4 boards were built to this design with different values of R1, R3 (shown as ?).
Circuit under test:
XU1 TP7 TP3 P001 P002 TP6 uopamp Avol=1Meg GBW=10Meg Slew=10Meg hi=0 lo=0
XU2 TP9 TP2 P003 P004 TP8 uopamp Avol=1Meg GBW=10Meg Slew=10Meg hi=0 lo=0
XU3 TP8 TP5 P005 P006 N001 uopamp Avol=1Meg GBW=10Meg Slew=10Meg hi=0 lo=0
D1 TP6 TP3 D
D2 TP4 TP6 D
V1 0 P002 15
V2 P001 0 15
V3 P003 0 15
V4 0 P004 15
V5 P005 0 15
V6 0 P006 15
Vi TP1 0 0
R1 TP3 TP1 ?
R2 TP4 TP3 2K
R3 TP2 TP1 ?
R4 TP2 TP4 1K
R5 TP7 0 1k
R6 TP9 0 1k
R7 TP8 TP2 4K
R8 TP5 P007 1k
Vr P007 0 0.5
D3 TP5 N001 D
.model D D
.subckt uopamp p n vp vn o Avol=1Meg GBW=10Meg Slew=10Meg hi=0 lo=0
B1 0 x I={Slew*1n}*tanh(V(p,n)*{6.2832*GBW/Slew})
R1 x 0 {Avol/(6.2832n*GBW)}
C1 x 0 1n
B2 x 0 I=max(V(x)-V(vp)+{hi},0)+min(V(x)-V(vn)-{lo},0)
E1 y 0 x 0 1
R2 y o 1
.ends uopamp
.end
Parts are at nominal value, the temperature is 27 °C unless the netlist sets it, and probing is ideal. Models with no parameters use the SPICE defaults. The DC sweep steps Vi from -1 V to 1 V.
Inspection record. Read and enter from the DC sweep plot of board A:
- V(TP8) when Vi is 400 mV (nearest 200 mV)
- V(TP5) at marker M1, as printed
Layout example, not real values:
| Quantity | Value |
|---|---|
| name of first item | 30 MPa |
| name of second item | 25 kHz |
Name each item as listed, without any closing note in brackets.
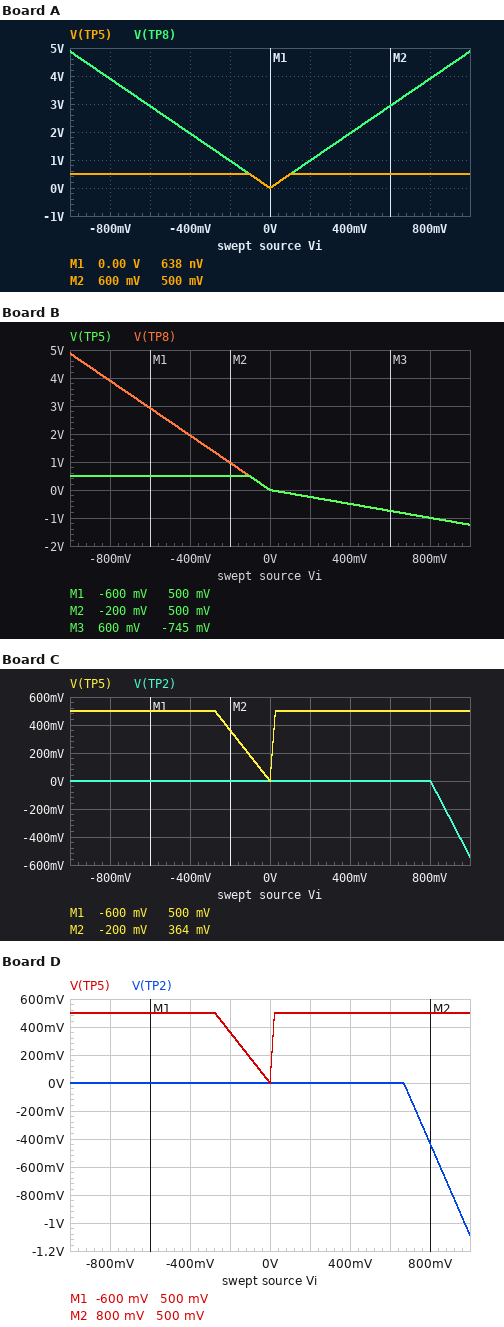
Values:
| Quantity | Value |
|---|---|
| V(TP8) when Vi is 400 mV | 2.0 V |
| V(TP5) at marker M1, as printed | 638 nV |
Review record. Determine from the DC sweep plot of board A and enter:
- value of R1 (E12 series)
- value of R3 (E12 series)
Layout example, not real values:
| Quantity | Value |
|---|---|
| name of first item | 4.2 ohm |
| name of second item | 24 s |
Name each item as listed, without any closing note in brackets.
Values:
| Quantity | Value |
|---|---|
| value of R1 | 820 Ω |
| value of R3 | 820 Ω |
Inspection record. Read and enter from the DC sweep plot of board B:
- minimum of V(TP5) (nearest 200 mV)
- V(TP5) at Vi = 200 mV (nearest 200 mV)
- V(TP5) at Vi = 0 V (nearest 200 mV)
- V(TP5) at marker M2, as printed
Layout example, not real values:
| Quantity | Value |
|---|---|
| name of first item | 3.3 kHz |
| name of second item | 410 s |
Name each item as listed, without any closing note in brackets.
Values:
| Quantity | Value |
|---|---|
| minimum of V(TP5) | -1.2 V |
| V(TP5) at Vi = 200 mV | -200 mV |
| V(TP5) at Vi = 0 V | 0 V |
| V(TP5) at marker M2, as printed | 500 mV |
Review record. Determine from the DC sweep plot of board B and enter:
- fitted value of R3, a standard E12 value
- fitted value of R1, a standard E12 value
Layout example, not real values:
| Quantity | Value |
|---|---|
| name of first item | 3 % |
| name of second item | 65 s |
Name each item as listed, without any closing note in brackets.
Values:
| Quantity | Value |
|---|---|
| fitted value of R3, a standard E12 value | 820 Ω |
| fitted value of R1, a standard E12 value | 2.2 kΩ |
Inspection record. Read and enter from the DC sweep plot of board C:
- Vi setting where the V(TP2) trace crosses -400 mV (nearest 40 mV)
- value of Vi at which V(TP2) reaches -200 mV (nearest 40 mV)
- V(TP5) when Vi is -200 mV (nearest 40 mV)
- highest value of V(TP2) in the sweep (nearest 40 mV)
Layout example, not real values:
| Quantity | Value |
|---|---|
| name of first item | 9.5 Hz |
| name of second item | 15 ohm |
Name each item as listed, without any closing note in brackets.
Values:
| Quantity | Value |
|---|---|
| Vi setting where the V(TP2) trace crosses -400 mV | 960 mV |
| value of Vi at which V(TP2) reaches -200 mV | 880 mV |
| V(TP5) when Vi is -200 mV | 360 mV |
| highest value of V(TP2) in the sweep | 0 V |
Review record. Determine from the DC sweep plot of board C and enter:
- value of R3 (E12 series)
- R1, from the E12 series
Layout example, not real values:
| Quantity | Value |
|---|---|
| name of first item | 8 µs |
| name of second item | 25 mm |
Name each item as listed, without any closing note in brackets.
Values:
| Quantity | Value |
|---|---|
| value of R3 | 2.2 kΩ |
| R1, from the E12 series | 390 Ω |
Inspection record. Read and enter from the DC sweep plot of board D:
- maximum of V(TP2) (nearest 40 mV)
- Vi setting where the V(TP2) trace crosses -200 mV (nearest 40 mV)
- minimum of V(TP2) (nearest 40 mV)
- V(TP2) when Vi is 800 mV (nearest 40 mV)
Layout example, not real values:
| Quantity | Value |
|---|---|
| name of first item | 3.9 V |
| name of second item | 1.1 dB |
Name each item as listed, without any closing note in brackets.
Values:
| Quantity | Value |
|---|---|
| maximum of V(TP2) | 0 V |
| Vi setting where the V(TP2) trace crosses -200 mV | 720 mV |
| minimum of V(TP2) | -1.08 V |
| V(TP2) when Vi is 800 mV | -440 mV |
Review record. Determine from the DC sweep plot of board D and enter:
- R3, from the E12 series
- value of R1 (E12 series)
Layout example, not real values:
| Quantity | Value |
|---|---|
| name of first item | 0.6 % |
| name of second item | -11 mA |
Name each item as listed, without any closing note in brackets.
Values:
| Quantity | Value |
|---|---|
| R3, from the E12 series | 2.2 kΩ |
| value of R1 | 330 Ω |
